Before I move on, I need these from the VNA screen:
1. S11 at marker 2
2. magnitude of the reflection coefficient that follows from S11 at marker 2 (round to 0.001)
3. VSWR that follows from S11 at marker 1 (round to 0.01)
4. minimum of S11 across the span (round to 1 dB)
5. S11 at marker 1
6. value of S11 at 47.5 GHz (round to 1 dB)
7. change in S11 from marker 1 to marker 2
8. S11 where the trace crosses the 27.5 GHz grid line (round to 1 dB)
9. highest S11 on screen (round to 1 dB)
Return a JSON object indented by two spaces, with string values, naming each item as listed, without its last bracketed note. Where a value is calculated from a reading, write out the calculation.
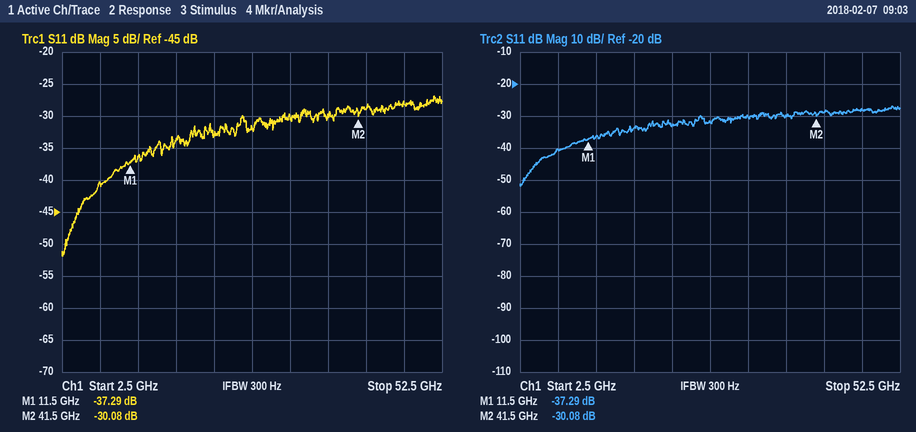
{
  "S11 at marker 2": "-30.08 dB",
  "magnitude of the reflection coefficient that follows from S11 at marker 2": "10^(-30.08/20) ≈ 0.031",
  "VSWR that follows from S11 at marker 1": "(1 + 0.0137)/(1 − 0.0137) ≈ 1.03",
  "minimum of S11 across the span": "-52 dB",
  "S11 at marker 1": "-37.29 dB",
  "value of S11 at 47.5 GHz": "-28 dB",
  "change in S11 from marker 1 to marker 2": "-30.08 − (-37.29) = 7.21 dB",
  "S11 where the trace crosses the 27.5 GHz grid line": "-32 dB",
  "highest S11 on screen": "-27 dB"
}
